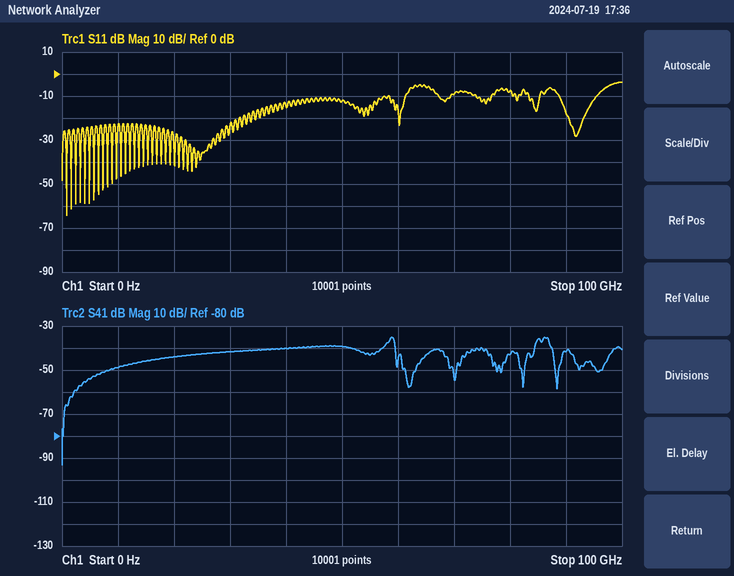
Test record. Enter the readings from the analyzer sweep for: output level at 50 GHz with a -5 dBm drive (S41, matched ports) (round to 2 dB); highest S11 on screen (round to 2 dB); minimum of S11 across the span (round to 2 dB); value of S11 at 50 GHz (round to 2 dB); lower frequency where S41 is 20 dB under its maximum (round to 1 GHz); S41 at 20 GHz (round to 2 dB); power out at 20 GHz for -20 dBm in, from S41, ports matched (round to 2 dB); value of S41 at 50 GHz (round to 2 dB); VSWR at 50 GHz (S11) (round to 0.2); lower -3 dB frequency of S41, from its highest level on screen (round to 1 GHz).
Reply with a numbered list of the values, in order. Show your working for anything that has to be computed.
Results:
1. -5 dBm + (-40 dB) = -44 dBm
2. -4 dB
3. -64 dB
4. -12 dB
5. 4 GHz
6. -44 dB
7. -20 dBm + (-44 dB) = -64 dBm
8. -40 dB
9. |Γ| = 10^(-12/20) = 0.2512; VSWR = (1 + 0.2512)/(1 − 0.2512) ≈ 1.67, so 1.6 to the nearest 0.2
10. 58 GHz
